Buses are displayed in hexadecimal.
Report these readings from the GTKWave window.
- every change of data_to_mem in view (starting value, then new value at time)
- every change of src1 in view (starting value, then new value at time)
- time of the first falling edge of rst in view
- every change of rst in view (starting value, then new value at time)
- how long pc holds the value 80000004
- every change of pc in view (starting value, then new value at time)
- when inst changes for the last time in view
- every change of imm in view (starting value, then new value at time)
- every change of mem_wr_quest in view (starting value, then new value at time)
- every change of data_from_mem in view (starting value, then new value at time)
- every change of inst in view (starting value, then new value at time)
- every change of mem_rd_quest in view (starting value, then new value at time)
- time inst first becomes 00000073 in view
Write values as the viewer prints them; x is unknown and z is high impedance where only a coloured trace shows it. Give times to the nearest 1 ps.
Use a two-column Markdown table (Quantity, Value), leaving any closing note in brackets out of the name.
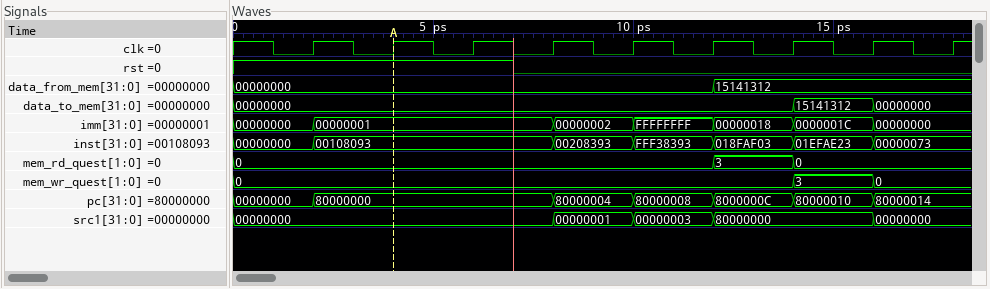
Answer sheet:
| Quantity | Value |
|---|---|
| every change of data_to_mem in view | 00000000, 15141312 at 14 ps, 00000000 at 16 ps |
| every change of src1 in view | 00000000, 00000001 at 8 ps, 00000003 at 10 ps, 80000000 at 12 ps, 00000000 at 16 ps |
| time of the first falling edge of rst in view | 7 ps |
| every change of rst in view | 1, 0 at 7 ps |
| how long pc holds the value 80000004 | 2 ps |
| every change of pc in view | 00000000, 80000000 at 2 ps, 80000004 at 8 ps, 80000008 at 10 ps, 8000000C at 12 ps, 80000010 at 14 ps, 80000014 at 16 ps |
| when inst changes for the last time in view | 16 ps |
| every change of imm in view | 00000000, 00000001 at 2 ps, 00000002 at 8 ps, FFFFFFFF at 10 ps, 00000018 at 12 ps, 0000001C at 14 ps, 00000000 at 16 ps |
| every change of mem_wr_quest in view | 0, 3 at 14 ps, 0 at 16 ps |
| every change of data_from_mem in view | 00000000, 15141312 at 12 ps |
| every change of inst in view | 00000000, 00108093 at 2 ps, 00208393 at 8 ps, FFF38393 at 10 ps, 018FAF03 at 12 ps, 01EFAE23 at 14 ps, 00000073 at 16 ps |
| every change of mem_rd_quest in view | 0, 3 at 12 ps, 0 at 14 ps |
| time inst first becomes 00000073 in view | 16 ps |
